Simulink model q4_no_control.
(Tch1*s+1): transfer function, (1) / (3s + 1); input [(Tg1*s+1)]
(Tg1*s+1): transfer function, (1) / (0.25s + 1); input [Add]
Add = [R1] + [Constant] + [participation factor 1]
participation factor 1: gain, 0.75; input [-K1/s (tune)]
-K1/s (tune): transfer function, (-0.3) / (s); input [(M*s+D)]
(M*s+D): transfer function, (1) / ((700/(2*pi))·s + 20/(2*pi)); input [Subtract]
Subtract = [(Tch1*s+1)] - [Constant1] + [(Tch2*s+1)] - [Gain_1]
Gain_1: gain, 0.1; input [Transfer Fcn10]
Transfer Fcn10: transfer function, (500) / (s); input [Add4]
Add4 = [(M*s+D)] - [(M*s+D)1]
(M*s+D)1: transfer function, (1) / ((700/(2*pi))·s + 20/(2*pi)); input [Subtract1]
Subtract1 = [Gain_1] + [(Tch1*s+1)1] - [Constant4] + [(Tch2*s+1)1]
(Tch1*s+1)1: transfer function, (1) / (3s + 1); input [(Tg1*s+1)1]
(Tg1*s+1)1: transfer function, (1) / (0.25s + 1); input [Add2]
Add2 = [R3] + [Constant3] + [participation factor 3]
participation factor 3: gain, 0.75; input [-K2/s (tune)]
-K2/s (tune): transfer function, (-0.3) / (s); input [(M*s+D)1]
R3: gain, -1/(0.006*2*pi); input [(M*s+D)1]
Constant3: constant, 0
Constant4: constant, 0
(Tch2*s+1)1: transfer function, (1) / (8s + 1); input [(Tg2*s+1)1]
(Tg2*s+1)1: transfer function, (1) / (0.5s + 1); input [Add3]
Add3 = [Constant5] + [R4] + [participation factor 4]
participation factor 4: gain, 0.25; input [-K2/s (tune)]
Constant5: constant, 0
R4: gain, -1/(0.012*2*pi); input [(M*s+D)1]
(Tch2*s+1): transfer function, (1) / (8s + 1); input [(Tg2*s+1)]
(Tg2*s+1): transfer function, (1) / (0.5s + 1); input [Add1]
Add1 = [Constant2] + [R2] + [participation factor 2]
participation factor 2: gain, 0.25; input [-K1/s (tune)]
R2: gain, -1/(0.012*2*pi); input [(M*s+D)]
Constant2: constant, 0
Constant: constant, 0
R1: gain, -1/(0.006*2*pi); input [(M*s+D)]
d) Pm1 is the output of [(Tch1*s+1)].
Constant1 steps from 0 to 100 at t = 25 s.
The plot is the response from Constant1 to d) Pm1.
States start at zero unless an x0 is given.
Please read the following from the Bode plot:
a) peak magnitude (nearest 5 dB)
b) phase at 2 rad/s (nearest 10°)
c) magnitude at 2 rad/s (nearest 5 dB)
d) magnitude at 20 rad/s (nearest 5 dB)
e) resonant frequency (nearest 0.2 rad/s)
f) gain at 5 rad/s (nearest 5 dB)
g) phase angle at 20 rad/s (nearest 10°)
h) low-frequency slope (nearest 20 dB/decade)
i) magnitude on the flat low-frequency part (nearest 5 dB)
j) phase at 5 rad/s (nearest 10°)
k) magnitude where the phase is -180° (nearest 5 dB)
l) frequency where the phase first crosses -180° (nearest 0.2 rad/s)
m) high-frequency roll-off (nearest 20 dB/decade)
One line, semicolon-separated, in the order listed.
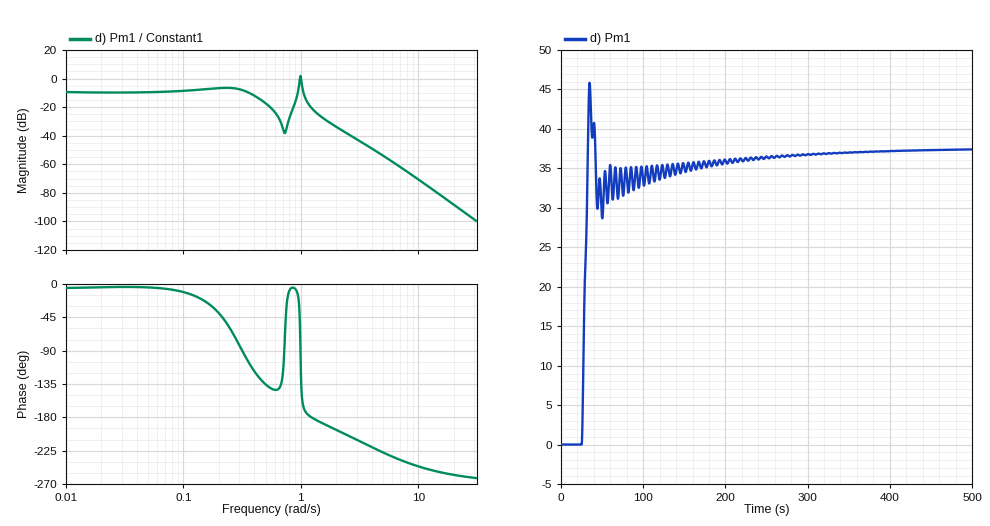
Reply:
0 dB; -200°; -35 dB; -90 dB; 1.0 rad/s; -55 dB; -260°; 0 dB/decade; -10 dB; -230°; -20 dB; 1.2 rad/s; -60 dB/decade
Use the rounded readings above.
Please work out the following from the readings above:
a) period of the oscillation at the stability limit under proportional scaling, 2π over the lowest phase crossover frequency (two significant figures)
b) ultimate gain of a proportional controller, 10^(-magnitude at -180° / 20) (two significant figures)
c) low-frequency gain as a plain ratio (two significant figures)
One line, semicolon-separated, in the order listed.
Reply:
5.2 s; 10; 0.32
